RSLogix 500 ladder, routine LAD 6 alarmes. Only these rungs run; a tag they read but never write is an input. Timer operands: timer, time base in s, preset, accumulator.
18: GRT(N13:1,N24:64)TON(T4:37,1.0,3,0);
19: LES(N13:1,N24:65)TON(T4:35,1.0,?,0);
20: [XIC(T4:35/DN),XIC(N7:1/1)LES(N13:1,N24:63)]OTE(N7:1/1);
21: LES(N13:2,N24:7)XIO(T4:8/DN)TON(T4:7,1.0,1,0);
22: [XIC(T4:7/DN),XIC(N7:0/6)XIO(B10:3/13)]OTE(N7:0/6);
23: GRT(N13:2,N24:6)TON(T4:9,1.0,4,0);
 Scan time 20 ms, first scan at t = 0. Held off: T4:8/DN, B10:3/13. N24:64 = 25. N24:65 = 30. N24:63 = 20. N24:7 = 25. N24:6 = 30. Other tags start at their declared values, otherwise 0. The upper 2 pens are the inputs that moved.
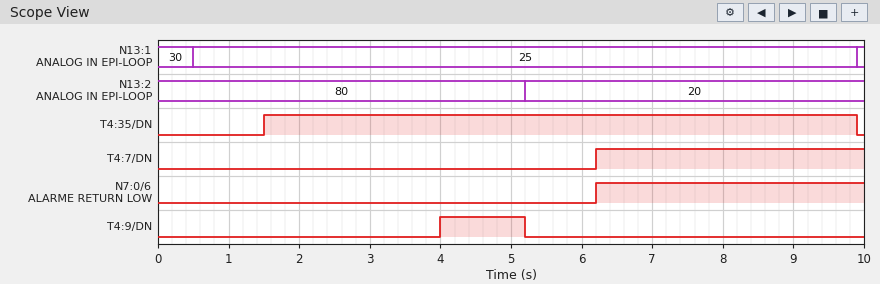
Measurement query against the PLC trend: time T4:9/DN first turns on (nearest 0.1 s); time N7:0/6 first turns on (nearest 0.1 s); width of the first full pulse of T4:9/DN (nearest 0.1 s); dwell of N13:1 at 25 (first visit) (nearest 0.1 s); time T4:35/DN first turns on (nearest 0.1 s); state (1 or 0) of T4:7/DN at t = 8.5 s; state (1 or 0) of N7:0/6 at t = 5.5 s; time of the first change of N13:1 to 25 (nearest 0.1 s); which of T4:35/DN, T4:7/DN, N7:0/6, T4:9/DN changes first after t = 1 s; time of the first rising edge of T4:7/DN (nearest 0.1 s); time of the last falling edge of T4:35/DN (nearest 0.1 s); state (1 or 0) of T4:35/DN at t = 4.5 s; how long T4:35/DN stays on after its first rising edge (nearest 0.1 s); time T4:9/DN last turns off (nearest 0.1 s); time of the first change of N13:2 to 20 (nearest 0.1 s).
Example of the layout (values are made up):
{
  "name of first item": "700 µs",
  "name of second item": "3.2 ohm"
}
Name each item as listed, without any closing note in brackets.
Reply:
{
  "time T4:9/DN first turns on": "4.0 s",
  "time N7:0/6 first turns on": "6.2 s",
  "width of the first full pulse of T4:9/DN": "1.2 s",
  "dwell of N13:1 at 25 (first visit)": "9.4 s",
  "time T4:35/DN first turns on": "1.5 s",
  "state (1 or 0) of T4:7/DN at t = 8.5 s": "1",
  "state (1 or 0) of N7:0/6 at t = 5.5 s": "0",
  "time of the first change of N13:1 to 25": "0.5 s",
  "which of T4:35/DN, T4:7/DN, N7:0/6, T4:9/DN changes first after t = 1 s": "T4:35/DN",
  "time of the first rising edge of T4:7/DN": "6.2 s",
  "time of the last falling edge of T4:35/DN": "9.9 s",
  "state (1 or 0) of T4:35/DN at t = 4.5 s": "1",
  "how long T4:35/DN stays on after its first rising edge": "8.4 s",
  "time T4:9/DN last turns off": "5.2 s",
  "time of the first change of N13:2 to 20": "5.2 s"
}
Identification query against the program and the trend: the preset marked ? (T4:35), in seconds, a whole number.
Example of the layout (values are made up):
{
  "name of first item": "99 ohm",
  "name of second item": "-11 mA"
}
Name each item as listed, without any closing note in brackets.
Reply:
{
  "the preset marked ? (T4:35), in seconds, a whole number": "1 s"
}
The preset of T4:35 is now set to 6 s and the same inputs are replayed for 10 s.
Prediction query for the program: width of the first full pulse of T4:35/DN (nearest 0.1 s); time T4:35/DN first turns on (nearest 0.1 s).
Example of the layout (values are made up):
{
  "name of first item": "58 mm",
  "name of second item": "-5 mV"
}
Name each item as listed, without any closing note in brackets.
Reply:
{
  "width of the first full pulse of T4:35/DN": "3.4 s",
  "time T4:35/DN first turns on": "6.5 s"
}
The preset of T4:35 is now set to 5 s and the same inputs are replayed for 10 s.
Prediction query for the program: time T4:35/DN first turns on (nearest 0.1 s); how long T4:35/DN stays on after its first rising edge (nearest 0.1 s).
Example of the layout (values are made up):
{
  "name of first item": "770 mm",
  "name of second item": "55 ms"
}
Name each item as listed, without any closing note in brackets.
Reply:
{
  "time T4:35/DN first turns on": "5.5 s",
  "how long T4:35/DN stays on after its first rising edge": "4.4 s"
}
